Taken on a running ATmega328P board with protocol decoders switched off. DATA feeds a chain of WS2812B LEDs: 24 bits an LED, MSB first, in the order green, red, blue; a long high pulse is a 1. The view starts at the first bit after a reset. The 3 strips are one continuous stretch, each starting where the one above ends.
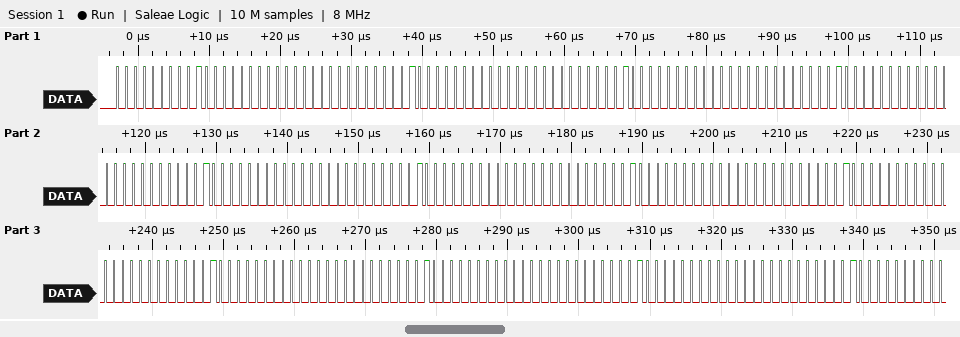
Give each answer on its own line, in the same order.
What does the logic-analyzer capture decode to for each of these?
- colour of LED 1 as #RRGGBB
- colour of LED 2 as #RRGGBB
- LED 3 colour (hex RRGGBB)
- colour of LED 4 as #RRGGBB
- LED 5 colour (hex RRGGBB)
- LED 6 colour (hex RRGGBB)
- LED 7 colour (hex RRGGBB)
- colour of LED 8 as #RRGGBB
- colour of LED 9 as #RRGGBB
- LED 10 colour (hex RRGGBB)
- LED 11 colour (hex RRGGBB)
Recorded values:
#400000
#400000
#400000
#400000
#400000
#400000
#400000
#400000
#400000
#400000
#400000
